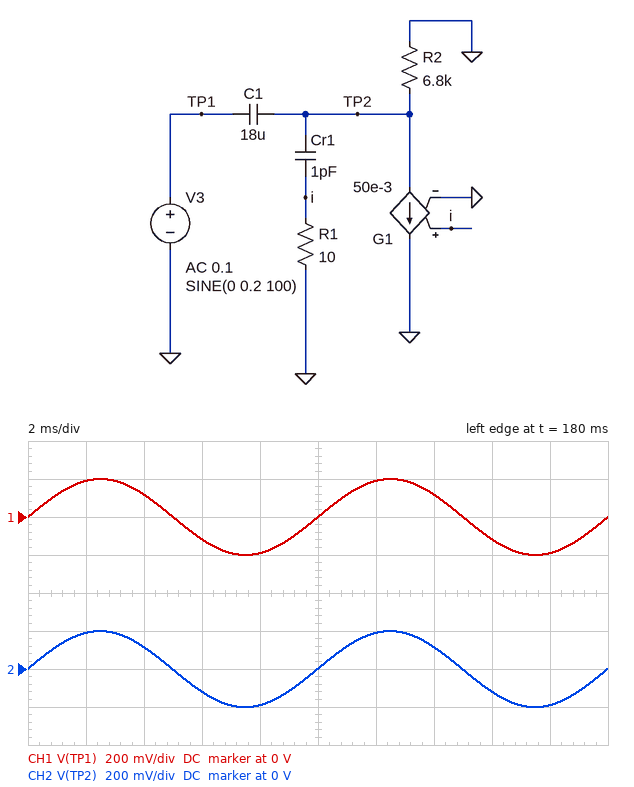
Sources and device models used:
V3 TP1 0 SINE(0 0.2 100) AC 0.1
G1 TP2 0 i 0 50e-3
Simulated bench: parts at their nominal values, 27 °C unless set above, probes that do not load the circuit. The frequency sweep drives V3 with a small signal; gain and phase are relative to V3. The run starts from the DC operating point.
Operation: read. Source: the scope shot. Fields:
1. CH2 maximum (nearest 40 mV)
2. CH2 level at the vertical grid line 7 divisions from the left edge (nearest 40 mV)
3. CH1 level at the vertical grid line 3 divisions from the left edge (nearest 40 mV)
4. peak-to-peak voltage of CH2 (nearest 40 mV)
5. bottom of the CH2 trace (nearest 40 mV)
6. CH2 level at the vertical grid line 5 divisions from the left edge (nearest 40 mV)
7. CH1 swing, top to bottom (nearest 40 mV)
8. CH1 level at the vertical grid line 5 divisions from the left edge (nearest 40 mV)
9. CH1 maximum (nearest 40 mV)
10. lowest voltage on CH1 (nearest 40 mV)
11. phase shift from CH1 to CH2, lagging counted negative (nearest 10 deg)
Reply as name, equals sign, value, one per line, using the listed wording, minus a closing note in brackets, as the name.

CH2 maximum = 200 mV
CH2 level at the vertical grid line 7 divisions from the left edge = 120 mV
CH1 level at the vertical grid line 3 divisions from the left edge = -120 mV
peak-to-peak voltage of CH2 = 400 mV
bottom of the CH2 trace = -200 mV
CH2 level at the vertical grid line 5 divisions from the left edge = 0 V
CH1 swing, top to bottom = 400 mV
CH1 level at the vertical grid line 5 divisions from the left edge = 0 V
CH1 maximum = 200 mV
lowest voltage on CH1 = -200 mV
phase shift from CH1 to CH2, lagging counted negative = 0 deg
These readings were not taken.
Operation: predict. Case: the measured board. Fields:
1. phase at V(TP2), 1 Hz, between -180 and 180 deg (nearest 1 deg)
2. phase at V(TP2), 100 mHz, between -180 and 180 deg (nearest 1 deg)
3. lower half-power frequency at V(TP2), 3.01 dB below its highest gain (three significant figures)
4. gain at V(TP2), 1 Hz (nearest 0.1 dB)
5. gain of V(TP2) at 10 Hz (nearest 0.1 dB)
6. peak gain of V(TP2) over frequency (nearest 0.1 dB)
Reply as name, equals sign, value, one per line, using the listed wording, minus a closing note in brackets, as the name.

phase at V(TP2), 1 Hz, between -180 and 180 deg = 52 deg
phase at V(TP2), 100 mHz, between -180 and 180 deg = 86 deg
lower half-power frequency at V(TP2), 3.01 dB below its highest gain = 1.30 Hz
gain at V(TP2), 1 Hz = -4.3 dB
gain of V(TP2) at 10 Hz = -0.1 dB
peak gain of V(TP2) over frequency = 0 dB
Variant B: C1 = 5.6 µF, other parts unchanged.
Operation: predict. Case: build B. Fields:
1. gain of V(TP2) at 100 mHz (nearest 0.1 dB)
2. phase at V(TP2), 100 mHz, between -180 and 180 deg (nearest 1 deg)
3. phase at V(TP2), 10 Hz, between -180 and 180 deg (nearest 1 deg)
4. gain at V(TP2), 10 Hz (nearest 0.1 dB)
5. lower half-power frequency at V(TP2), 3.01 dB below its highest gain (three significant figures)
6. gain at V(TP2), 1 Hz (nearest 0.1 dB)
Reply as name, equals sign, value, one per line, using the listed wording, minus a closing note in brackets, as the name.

gain of V(TP2) at 100 mHz = -32.4 dB
phase at V(TP2), 100 mHz, between -180 and 180 deg = 89 deg
phase at V(TP2), 10 Hz, between -180 and 180 deg = 23 deg
gain at V(TP2), 10 Hz = -0.7 dB
lower half-power frequency at V(TP2), 3.01 dB below its highest gain = 4.18 Hz
gain at V(TP2), 1 Hz = -12.7 dB
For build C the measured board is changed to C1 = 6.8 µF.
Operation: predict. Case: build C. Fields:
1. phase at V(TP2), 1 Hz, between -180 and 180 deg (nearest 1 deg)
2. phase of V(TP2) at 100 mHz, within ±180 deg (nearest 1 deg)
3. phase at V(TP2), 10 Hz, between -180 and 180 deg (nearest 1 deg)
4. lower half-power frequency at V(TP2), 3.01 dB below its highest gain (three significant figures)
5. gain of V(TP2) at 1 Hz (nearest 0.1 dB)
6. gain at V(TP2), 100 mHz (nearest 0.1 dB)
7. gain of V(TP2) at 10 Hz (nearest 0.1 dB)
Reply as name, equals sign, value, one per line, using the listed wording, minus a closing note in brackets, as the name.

phase at V(TP2), 1 Hz, between -180 and 180 deg = 74 deg
phase of V(TP2) at 100 mHz, within ±180 deg = 88 deg
phase at V(TP2), 10 Hz, between -180 and 180 deg = 19 deg
lower half-power frequency at V(TP2), 3.01 dB below its highest gain = 3.44 Hz
gain of V(TP2) at 1 Hz = -11.1 dB
gain at V(TP2), 100 mHz = -30.7 dB
gain of V(TP2) at 10 Hz = -0.5 dB
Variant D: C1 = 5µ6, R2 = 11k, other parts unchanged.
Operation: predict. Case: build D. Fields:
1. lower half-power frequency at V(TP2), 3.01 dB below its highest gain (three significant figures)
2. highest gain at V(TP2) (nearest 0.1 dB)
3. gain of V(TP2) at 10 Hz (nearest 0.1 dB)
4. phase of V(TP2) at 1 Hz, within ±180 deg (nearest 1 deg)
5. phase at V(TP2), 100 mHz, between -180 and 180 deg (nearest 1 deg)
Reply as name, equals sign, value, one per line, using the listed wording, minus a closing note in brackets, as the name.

lower half-power frequency at V(TP2), 3.01 dB below its highest gain = 2.58 Hz
highest gain at V(TP2) = 0 dB
gain of V(TP2) at 10 Hz = -0.3 dB
phase of V(TP2) at 1 Hz, within ±180 deg = 69 deg
phase at V(TP2), 100 mHz, between -180 and 180 deg = 88 deg
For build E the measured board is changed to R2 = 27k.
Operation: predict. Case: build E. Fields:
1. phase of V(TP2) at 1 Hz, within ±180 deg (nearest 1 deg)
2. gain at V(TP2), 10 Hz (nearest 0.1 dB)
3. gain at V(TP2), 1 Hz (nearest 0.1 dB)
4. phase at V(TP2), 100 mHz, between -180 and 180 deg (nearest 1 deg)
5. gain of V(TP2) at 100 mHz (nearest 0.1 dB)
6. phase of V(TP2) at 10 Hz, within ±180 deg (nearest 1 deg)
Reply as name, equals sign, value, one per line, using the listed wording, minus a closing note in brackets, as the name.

phase of V(TP2) at 1 Hz, within ±180 deg = 18 deg
gain at V(TP2), 10 Hz = 0 dB
gain at V(TP2), 1 Hz = -0.4 dB
phase at V(TP2), 100 mHz, between -180 and 180 deg = 73 deg
gain of V(TP2) at 100 mHz = -10.7 dB
phase of V(TP2) at 10 Hz, within ±180 deg = 2 deg
